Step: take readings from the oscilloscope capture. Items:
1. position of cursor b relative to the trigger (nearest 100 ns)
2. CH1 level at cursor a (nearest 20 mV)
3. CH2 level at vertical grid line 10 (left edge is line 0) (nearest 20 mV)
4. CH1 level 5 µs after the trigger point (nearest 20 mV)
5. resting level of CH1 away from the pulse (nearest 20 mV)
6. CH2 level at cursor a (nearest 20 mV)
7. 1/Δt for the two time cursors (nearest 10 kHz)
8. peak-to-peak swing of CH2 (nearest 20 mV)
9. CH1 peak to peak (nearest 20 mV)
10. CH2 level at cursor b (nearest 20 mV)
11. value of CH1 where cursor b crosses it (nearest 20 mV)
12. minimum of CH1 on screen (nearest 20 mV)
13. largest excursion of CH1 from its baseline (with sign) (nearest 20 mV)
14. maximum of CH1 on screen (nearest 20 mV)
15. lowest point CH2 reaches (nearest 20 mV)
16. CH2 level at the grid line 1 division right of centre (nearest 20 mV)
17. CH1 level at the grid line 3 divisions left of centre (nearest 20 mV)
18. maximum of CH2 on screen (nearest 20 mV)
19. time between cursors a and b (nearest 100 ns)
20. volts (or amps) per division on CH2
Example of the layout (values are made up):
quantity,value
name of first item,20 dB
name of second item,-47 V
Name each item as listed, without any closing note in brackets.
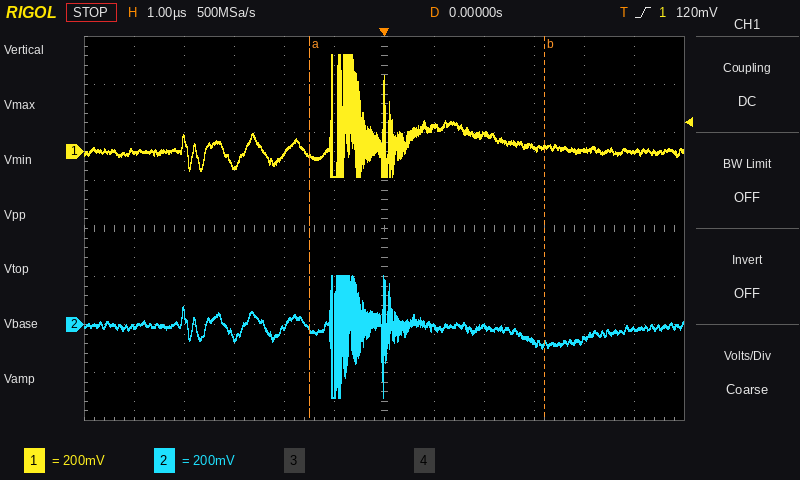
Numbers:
quantity,value
position of cursor b relative to the trigger,+3.2 µs
CH1 level at cursor a,-20 mV
CH2 level at vertical grid line 10 (left edge is line 0),-60 mV
CH1 level 5 µs after the trigger point,0 mV
resting level of CH1 away from the pulse,0 mV
CH2 level at cursor a,-20 mV
1/Δt for the two time cursors,210 kHz
peak-to-peak swing of CH2,500 mV
CH1 peak to peak,500 mV
CH2 level at cursor b,-80 mV
value of CH1 where cursor b crosses it,20 mV
minimum of CH1 on screen,-100 mV
largest excursion of CH1 from its baseline (with sign),+400 mV
maximum of CH1 on screen,400 mV
lowest point CH2 reaches,-300 mV
CH2 level at the grid line 1 division right of centre,-20 mV
CH1 level at the grid line 3 divisions left of centre,-60 mV
maximum of CH2 on screen,200 mV
time between cursors a and b,4.7 µs
volts (or amps) per division on CH2,200 mV
